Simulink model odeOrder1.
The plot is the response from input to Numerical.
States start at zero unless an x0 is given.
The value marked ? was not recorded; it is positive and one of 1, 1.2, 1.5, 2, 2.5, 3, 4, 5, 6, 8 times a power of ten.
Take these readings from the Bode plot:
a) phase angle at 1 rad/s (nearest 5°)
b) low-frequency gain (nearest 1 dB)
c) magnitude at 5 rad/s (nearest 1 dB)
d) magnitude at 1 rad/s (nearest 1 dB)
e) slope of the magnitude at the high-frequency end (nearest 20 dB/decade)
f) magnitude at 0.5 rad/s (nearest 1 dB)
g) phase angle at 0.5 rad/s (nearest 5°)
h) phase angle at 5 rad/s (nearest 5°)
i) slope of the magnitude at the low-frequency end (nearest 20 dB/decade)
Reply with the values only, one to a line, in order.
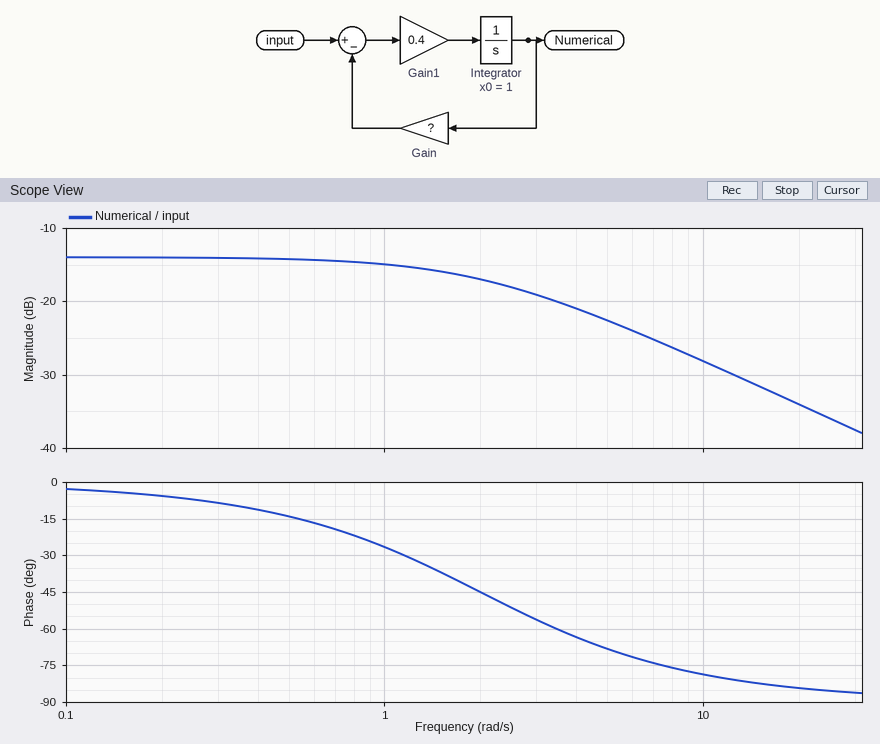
-25°
-14 dB
-23 dB
-15 dB
-20 dB/decade
-14 dB
-15°
-70°
0 dB/decade
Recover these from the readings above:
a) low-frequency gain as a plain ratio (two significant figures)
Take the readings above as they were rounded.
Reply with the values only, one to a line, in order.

0.20
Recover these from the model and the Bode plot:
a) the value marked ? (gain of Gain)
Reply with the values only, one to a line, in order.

5
